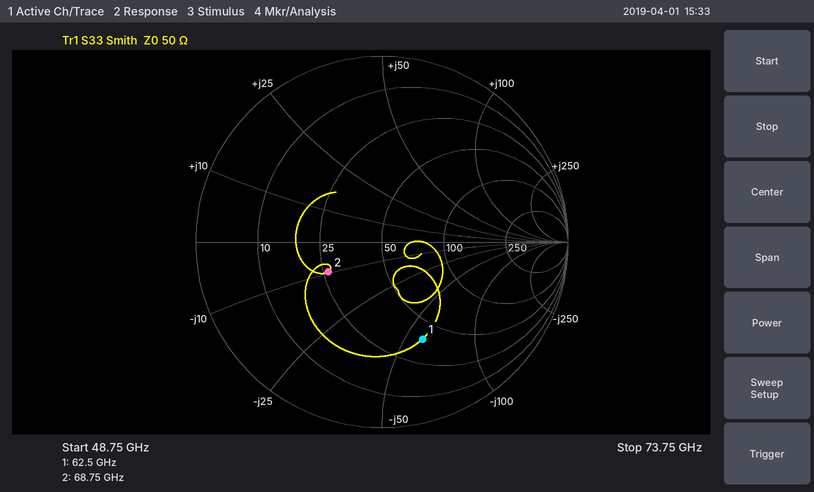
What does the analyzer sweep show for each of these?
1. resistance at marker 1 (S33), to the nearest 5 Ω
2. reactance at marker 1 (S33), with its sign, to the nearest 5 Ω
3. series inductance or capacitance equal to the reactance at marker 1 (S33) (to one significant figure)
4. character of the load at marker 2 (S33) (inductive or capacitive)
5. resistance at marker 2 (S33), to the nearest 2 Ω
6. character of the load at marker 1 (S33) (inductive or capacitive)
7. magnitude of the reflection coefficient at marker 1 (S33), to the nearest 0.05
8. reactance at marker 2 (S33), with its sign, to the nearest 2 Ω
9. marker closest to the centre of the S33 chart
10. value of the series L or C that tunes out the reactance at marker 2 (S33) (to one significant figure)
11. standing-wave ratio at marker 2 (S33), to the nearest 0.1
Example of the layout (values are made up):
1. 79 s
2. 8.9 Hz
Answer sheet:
1. 40 Ω
2. -60 Ω
3. 40 fF
4. capacitive
5. 26 Ω
6. capacitive
7. 0.55
8. -10 Ω
9. marker 2
10. 20 pH
11. 2.0
